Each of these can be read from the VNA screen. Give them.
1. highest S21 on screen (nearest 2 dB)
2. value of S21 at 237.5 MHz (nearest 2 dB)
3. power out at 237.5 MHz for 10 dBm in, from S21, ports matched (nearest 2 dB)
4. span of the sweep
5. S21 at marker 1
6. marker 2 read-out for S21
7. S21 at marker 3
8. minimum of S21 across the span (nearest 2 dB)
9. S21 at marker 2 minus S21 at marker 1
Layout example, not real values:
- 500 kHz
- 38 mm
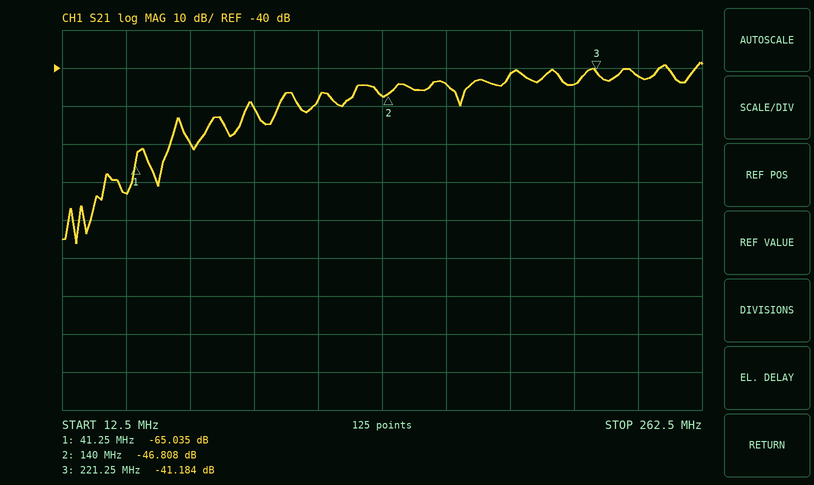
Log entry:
- -38 dB
- -42 dB
- -32 dBm
- 250 MHz
- -65.035 dB
- -46.808 dB
- -41.184 dB
- -86 dB
- 18.227 dB
